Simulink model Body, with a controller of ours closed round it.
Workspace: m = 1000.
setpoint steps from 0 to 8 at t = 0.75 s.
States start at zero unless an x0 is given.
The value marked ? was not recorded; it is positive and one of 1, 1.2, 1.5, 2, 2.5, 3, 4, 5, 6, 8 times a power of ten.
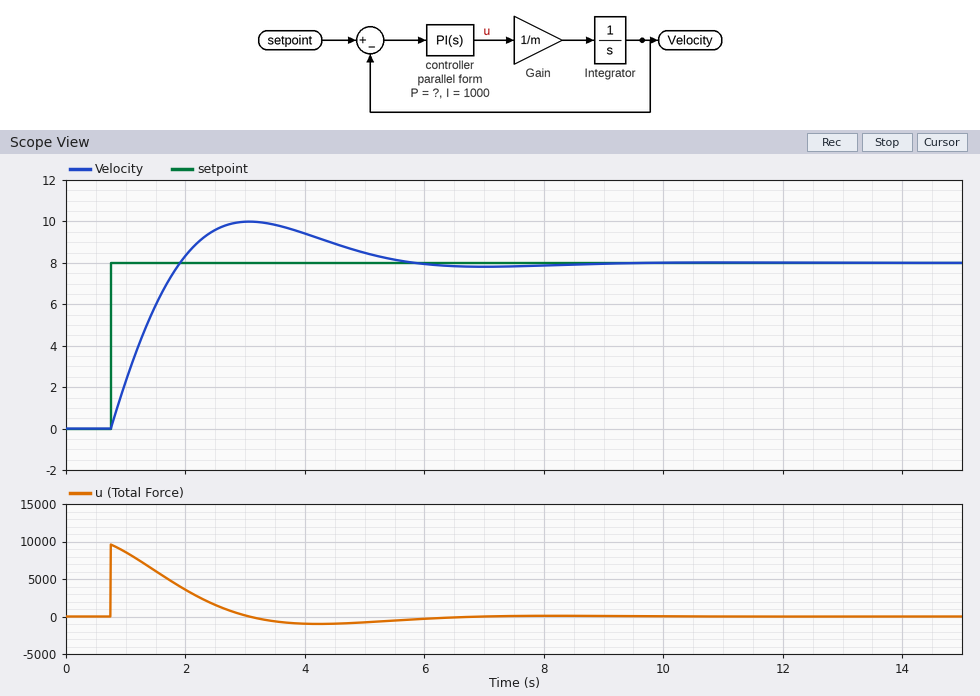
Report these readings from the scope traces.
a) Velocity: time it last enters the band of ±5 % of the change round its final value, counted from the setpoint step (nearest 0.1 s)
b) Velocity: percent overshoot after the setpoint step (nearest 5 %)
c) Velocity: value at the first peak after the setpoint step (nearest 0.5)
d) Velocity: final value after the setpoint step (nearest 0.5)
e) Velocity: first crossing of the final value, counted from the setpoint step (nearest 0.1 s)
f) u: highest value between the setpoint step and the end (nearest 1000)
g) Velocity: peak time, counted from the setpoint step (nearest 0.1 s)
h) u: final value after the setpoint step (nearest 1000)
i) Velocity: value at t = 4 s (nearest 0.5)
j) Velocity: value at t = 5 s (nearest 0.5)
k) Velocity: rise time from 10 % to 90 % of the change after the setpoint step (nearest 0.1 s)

4.4 s
25 %
10.0
8.0
1.2 s
10000
2.3 s
0
9.5
8.5
0.9 s
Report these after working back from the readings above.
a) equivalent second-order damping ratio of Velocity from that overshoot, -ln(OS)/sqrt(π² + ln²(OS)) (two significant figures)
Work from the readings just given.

0.40
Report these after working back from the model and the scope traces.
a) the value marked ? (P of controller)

1200
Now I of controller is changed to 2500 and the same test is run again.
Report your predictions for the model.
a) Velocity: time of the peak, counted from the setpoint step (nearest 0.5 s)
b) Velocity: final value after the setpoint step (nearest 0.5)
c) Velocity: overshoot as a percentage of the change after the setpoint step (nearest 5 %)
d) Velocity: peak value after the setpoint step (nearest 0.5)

1.5 s
8.0
40 %
11.0
